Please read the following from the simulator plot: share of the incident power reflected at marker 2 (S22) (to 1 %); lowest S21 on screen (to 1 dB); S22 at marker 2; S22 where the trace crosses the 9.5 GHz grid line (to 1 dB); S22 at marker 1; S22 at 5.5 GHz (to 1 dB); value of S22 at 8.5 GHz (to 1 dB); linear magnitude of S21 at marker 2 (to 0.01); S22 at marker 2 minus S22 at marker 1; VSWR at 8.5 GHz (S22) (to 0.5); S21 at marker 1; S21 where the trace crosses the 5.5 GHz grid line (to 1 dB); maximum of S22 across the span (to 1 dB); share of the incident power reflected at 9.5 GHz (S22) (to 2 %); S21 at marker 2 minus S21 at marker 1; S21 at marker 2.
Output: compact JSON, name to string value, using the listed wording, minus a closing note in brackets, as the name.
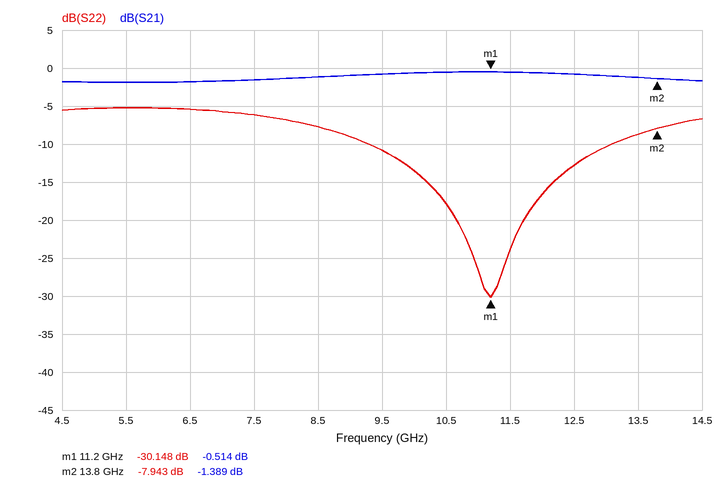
{"share of the incident power reflected at marker 2 (S22)": "16 %", "lowest S21 on screen": "-2 dB", "S22 at marker 2": "-7.943 dB", "S22 where the trace crosses the 9.5 GHz grid line": "-11 dB", "S22 at marker 1": "-30.148 dB", "S22 at 5.5 GHz": "-5 dB", "value of S22 at 8.5 GHz": "-8 dB", "linear magnitude of S21 at marker 2": "0.85", "S22 at marker 2 minus S22 at marker 1": "22.205 dB", "VSWR at 8.5 GHz (S22)": "2.5", "S21 at marker 1": "-0.514 dB", "S21 where the trace crosses the 5.5 GHz grid line": "-2 dB", "maximum of S22 across the span": "-5 dB", "share of the incident power reflected at 9.5 GHz (S22)": "8 %", "S21 at marker 2 minus S21 at marker 1": "-0.875 dB", "S21 at marker 2": "-1.389 dB"}
